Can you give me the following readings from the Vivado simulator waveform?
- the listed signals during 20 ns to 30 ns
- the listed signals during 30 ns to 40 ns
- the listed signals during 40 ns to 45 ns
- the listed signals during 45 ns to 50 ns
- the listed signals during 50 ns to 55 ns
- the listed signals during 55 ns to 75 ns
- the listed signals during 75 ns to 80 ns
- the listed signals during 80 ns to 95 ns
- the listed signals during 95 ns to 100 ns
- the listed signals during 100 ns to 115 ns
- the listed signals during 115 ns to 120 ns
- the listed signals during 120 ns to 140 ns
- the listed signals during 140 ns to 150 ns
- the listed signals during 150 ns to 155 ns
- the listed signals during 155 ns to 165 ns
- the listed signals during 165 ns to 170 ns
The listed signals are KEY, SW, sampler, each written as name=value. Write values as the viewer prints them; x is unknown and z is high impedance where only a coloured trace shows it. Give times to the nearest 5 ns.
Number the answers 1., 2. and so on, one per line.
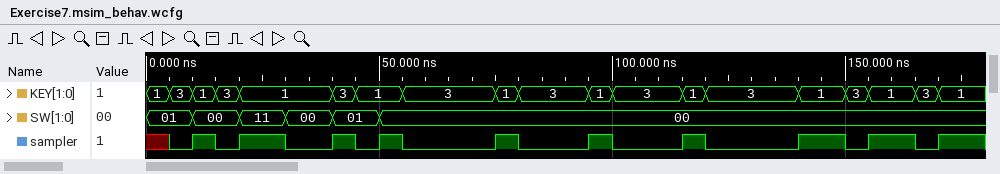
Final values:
1. KEY=1, SW=11, sampler=1
2. KEY=1, SW=00, sampler=0
3. KEY=3, SW=01, sampler=1
4. KEY=1, SW=01, sampler=0
5. KEY=1, SW=00, sampler=1
6. KEY=3, SW=00, sampler=0
7. KEY=1, SW=00, sampler=1
8. KEY=3, SW=00, sampler=0
9. KEY=1, SW=00, sampler=1
10. KEY=3, SW=00, sampler=0
11. KEY=1, SW=00, sampler=1
12. KEY=3, SW=00, sampler=0
13. KEY=1, SW=00, sampler=1
14. KEY=3, SW=00, sampler=0
15. KEY=1, SW=00, sampler=1
16. KEY=3, SW=00, sampler=0
